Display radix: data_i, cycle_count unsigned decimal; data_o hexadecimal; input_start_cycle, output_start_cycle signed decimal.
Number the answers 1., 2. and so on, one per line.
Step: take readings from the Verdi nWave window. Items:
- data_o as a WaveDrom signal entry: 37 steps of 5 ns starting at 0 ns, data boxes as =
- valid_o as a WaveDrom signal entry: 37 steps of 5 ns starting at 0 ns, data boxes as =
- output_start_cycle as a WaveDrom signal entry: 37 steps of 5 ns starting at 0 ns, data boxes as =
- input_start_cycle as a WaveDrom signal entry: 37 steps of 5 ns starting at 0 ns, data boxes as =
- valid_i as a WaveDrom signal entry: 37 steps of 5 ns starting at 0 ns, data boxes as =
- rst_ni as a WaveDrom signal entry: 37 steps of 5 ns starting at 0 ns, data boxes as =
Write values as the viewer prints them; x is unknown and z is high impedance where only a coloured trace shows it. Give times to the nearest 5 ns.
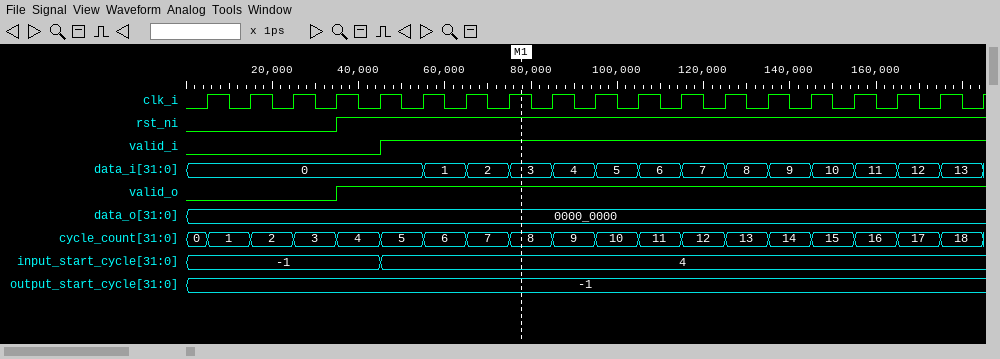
1. {name: 'data_o', wave: '=....................................', data: '0000_0000'}
2. {name: 'valid_o', wave: '0......1.............................'}
3. {name: 'output_start_cycle', wave: '=....................................', data: '-1'}
4. {name: 'input_start_cycle', wave: '=........=...........................', data: '-1 4'}
5. {name: 'valid_i', wave: '0........1...........................'}
6. {name: 'rst_ni', wave: '0......1.............................'}
